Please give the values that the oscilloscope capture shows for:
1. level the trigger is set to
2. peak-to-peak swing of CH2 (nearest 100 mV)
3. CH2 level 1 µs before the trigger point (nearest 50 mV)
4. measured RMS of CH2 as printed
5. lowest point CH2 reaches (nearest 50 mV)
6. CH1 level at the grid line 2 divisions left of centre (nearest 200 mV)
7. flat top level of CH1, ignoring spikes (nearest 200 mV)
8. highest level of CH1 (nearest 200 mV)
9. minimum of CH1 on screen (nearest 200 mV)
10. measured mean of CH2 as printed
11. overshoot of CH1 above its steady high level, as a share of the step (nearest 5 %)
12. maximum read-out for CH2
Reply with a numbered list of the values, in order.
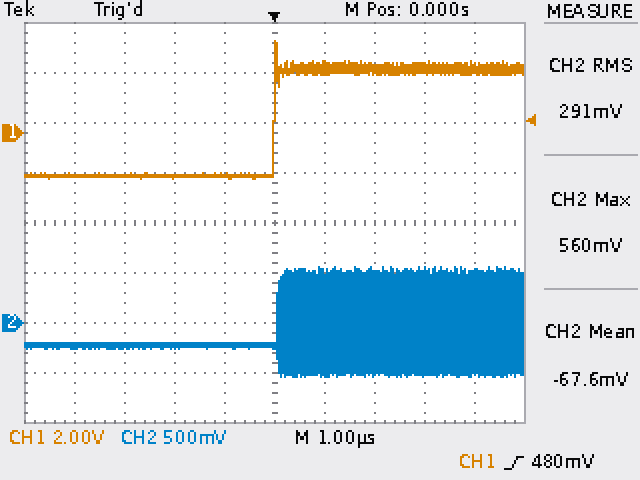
1. 480 mV
2. 1.10 V
3. -200 mV
4. 291 mV
5. -550 mV
6. -1.8 V
7. 2.6 V
8. 3.6 V
9. -1.8 V
10. -67.6 mV
11. 25 %
12. 560 mV
